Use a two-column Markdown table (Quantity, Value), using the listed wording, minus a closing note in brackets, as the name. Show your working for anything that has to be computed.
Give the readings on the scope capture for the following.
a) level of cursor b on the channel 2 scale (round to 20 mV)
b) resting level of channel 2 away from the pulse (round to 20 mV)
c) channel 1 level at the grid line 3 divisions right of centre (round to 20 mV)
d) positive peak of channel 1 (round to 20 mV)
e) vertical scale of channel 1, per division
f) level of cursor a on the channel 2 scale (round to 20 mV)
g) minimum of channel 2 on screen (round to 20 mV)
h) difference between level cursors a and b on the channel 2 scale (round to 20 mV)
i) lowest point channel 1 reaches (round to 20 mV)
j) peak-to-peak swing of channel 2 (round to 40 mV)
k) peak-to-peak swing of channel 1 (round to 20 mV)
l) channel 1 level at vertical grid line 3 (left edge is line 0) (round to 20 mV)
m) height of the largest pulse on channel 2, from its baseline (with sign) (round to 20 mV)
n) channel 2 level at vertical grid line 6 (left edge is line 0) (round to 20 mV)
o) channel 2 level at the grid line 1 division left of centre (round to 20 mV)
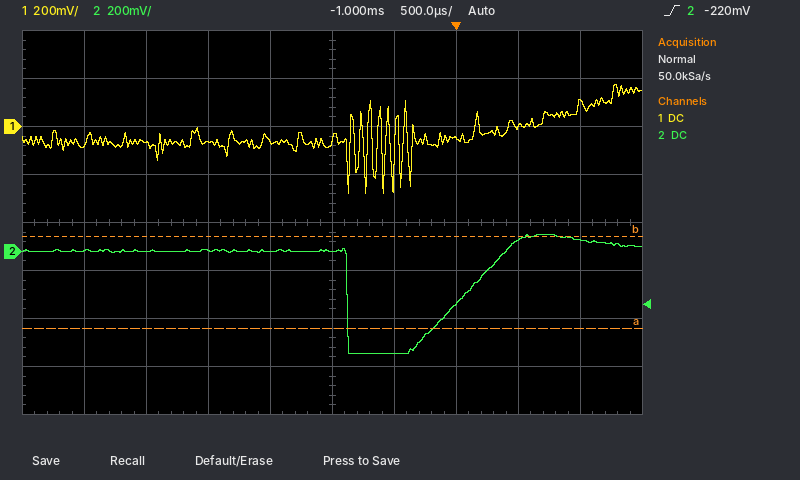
| Quantity | Value |
|---|---|
| level of cursor b on the channel 2 scale | 60 mV |
| resting level of channel 2 away from the pulse | 0 mV |
| channel 1 level at the grid line 3 divisions right of centre | 0 mV |
| positive peak of channel 1 | 180 mV |
| vertical scale of channel 1, per division | 200 mV |
| level of cursor a on the channel 2 scale | -320 mV |
| minimum of channel 2 on screen | -420 mV |
| difference between level cursors a and b on the channel 2 scale | 380 mV |
| lowest point channel 1 reaches | -280 mV |
| peak-to-peak swing of channel 2 | 480 mV |
| peak-to-peak swing of channel 1 | 180 mV − (-280 mV) = 460 mV |
| channel 1 level at vertical grid line 3 (left edge is line 0) | -60 mV |
| height of the largest pulse on channel 2, from its baseline (with sign) | -420 mV − (0 mV) = -420 mV |
| channel 2 level at vertical grid line 6 (left edge is line 0) | -420 mV |
| channel 2 level at the grid line 1 division left of centre | 0 mV |
